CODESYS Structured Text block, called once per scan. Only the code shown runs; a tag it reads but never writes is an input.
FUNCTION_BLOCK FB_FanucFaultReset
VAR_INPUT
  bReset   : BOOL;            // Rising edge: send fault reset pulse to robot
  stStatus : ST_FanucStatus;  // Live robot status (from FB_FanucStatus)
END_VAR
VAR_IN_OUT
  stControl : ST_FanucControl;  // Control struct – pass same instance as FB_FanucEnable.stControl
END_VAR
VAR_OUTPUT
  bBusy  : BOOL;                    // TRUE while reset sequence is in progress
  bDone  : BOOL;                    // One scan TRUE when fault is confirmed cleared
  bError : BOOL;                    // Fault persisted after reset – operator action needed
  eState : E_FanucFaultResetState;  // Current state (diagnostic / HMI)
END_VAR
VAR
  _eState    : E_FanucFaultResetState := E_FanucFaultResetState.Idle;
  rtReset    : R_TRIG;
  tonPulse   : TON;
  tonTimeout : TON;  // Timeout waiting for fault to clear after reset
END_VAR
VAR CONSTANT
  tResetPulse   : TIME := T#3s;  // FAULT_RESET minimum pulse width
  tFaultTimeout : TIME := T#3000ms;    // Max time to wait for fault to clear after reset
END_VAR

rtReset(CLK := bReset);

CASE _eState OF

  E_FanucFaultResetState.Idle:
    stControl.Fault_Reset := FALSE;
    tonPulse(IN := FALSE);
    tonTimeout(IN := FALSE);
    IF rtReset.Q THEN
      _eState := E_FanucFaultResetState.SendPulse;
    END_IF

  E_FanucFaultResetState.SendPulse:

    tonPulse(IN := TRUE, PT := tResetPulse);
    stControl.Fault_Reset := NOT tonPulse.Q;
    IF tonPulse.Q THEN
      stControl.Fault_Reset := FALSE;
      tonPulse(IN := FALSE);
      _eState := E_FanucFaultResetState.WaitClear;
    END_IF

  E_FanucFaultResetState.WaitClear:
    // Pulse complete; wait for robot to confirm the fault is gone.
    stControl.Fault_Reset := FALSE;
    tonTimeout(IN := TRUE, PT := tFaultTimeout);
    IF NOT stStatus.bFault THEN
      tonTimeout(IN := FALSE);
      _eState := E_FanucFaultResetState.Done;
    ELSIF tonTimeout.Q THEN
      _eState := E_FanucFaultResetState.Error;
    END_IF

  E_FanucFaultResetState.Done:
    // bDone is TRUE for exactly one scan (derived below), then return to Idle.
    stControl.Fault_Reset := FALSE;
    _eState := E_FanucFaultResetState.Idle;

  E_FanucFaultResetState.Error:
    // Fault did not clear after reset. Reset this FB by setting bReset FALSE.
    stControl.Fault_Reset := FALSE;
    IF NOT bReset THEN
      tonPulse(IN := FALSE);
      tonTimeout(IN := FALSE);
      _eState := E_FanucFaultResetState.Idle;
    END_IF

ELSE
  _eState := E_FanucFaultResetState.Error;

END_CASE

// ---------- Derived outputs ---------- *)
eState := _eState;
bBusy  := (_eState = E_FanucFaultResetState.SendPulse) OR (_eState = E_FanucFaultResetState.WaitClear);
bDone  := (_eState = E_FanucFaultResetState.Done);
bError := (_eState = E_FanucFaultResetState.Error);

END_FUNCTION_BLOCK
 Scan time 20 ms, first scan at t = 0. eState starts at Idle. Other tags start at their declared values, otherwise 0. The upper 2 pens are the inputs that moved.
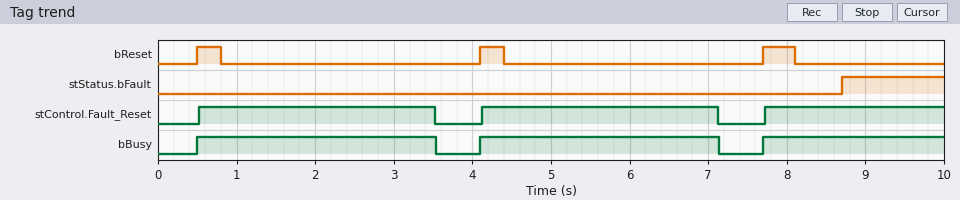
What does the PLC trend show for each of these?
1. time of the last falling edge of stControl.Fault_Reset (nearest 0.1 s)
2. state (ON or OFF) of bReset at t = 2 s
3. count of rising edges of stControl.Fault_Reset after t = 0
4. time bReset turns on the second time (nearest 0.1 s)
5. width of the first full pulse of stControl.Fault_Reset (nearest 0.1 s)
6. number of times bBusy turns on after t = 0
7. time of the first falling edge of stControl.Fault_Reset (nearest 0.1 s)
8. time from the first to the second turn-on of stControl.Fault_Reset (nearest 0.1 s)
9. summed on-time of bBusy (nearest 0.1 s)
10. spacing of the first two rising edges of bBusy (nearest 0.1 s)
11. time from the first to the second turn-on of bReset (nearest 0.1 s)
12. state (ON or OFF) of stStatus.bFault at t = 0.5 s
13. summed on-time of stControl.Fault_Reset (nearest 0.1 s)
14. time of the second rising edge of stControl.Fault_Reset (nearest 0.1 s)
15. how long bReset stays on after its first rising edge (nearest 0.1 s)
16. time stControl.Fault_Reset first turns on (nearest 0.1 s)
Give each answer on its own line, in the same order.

7.1 s
OFF
3
4.1 s
3.0 s
3
3.5 s
3.6 s
8.4 s
3.6 s
3.6 s
OFF
8.3 s
4.1 s
0.3 s
0.5 s
